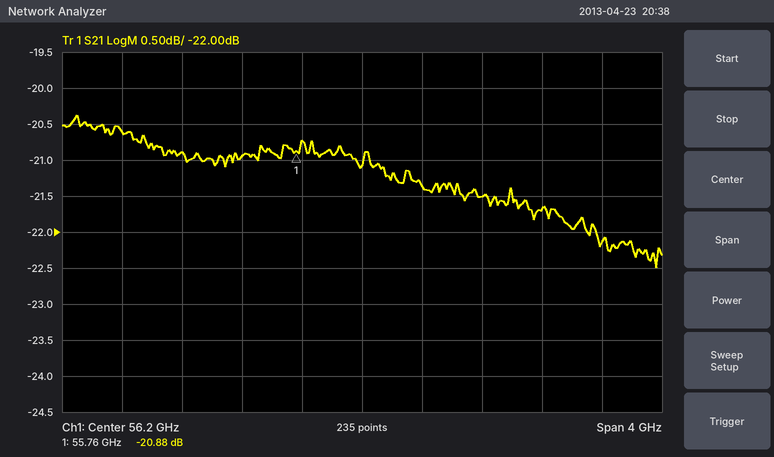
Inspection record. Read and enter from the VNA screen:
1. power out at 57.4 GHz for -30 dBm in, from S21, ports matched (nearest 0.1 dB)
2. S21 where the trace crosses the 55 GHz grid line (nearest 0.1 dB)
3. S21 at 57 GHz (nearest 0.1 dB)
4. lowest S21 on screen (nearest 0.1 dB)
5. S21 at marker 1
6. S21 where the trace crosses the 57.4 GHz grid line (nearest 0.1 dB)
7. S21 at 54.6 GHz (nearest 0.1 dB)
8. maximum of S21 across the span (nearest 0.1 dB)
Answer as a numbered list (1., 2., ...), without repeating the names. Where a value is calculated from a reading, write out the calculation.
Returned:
1. -30 dBm + (-21.7 dB) = -51.7 dBm
2. -20.9 dB
3. -21.5 dB
4. -22.5 dB
5. -20.88 dB
6. -21.7 dB
7. -20.6 dB
8. -20.4 dB
